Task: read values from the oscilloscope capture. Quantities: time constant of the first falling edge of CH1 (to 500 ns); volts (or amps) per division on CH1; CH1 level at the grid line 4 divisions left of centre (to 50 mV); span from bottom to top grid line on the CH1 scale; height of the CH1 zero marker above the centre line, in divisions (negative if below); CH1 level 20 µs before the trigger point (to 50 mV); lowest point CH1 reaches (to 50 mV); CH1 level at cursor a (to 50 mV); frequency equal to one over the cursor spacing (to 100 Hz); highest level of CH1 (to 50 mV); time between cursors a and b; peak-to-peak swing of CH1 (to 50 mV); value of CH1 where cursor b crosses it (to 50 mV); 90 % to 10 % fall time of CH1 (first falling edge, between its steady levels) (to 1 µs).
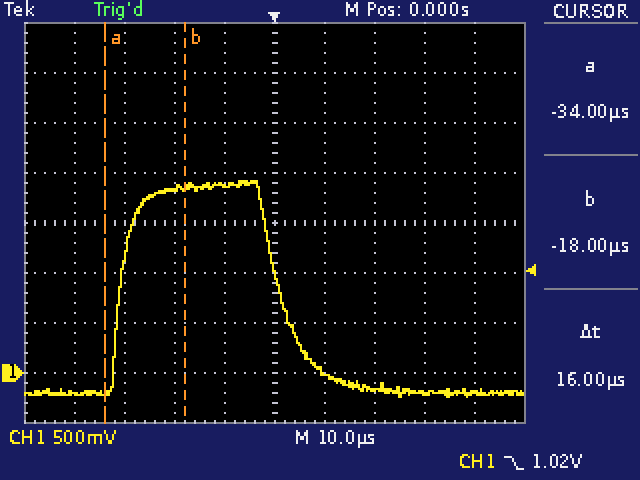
5.5 µs
500 mV
-200 mV
4 V
-3.0 div
1.85 V
-250 mV
-200 mV
62.5 kHz
1.90 V
16 µs
2.15 V
1.85 V
12 µs
